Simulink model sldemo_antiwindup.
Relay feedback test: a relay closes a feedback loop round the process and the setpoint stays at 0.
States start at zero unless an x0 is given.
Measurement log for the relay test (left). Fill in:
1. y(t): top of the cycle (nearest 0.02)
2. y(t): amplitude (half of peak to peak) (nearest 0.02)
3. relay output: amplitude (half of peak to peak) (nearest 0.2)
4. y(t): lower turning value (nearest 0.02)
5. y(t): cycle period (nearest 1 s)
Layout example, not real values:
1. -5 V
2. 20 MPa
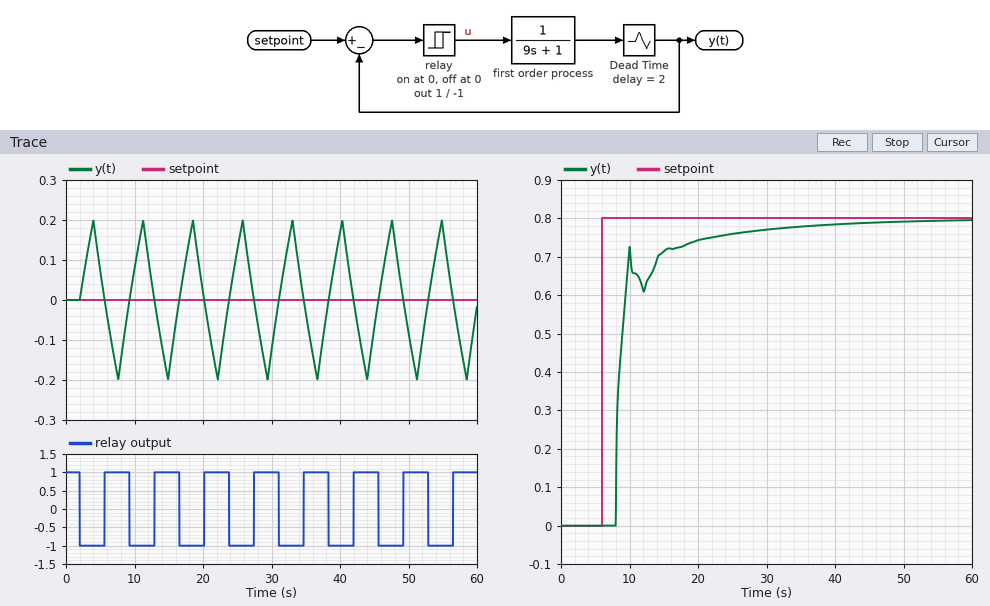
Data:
1. 0.20
2. 0.20
3. 1.0
4. -0.20
5. 7 s
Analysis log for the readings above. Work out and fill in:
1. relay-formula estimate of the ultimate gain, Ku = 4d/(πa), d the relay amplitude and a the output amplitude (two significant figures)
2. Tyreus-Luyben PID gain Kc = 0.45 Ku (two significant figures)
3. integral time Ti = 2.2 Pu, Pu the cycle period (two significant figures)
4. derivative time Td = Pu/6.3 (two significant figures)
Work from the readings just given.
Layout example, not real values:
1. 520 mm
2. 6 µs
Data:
1. 6.4
2. 2.9
3. 15 s
4. 1.1 s
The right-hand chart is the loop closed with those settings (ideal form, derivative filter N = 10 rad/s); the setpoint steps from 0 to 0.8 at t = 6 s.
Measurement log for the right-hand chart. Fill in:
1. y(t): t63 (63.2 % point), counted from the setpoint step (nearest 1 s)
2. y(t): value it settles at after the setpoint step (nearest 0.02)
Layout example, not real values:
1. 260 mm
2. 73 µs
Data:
1. 3 s
2. 0.80
